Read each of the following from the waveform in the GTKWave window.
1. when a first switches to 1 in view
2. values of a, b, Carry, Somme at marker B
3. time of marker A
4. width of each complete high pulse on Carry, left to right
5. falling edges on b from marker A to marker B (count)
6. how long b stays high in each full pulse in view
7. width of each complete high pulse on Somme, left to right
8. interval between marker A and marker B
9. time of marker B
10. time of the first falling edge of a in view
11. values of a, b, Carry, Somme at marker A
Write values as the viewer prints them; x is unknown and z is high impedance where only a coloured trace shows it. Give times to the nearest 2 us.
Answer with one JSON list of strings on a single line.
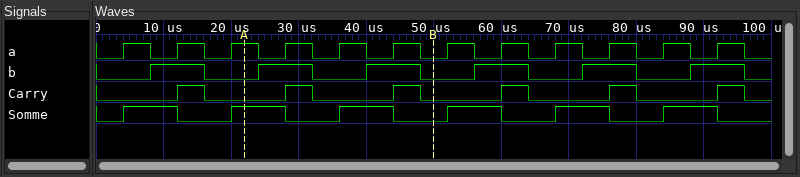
["4 us", "a=0, b=0, Carry=0, Somme=0", "22 us", "4 us, 4 us, 4 us, 4 us, 4 us, 4 us", "2", "8 us, 8 us, 8 us, 8 us, 8 us, 8 us", "8 us, 8 us, 8 us, 8 us, 8 us, 8 us", "28 us", "50 us", "8 us", "a=1, b=0, Carry=0, Somme=1"]
